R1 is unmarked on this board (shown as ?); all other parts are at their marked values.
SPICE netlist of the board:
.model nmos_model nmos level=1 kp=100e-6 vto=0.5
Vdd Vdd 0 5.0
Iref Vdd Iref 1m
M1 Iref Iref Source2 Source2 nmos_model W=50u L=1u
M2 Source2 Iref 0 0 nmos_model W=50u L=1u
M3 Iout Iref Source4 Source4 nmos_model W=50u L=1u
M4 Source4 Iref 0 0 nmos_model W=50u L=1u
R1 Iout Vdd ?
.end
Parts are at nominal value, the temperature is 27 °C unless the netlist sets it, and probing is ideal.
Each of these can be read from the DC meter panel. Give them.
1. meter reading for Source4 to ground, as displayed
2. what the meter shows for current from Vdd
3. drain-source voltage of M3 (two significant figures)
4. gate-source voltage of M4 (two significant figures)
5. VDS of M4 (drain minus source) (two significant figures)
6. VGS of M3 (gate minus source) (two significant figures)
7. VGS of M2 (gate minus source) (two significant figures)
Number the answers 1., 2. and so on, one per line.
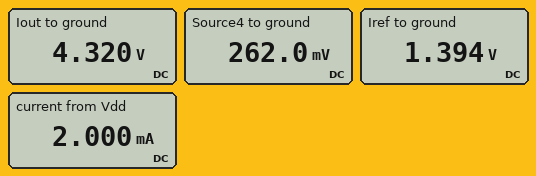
1. 262.0 mV
2. 2.000 mA
3. 4.1 V
4. 1.4 V
5. 260 mV
6. 1.1 V
7. 1.4 V
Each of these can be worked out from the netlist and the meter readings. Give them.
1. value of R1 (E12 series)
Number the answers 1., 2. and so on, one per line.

1. 680 Ω
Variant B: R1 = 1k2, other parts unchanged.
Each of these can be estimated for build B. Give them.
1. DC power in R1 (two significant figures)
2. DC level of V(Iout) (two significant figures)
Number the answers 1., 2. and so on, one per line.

1. 1.2 mW
2. 3.8 V
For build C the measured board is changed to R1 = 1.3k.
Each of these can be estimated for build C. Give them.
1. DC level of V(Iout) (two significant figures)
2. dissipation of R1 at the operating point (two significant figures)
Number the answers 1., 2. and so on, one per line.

1. 3.7 V
2. 1.3 mW
